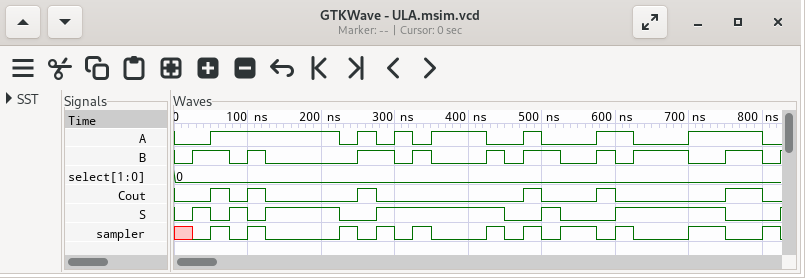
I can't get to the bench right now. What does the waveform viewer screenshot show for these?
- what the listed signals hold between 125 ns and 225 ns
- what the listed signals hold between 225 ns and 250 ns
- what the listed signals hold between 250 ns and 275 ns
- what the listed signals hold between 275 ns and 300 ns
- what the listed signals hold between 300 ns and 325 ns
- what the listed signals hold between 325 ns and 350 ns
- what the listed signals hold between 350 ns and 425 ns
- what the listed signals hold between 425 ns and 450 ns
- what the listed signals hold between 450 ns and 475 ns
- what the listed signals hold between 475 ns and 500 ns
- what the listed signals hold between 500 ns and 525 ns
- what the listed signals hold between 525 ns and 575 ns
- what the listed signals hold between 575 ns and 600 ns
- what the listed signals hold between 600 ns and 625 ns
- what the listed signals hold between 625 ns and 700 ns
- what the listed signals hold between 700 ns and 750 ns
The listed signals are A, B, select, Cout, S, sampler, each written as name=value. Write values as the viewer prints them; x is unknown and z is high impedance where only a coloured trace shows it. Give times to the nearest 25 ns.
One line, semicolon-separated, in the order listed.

A=1, B=0, select=0, Cout=0, S=1, sampler=0; A=0, B=0, select=0, Cout=0, S=0, sampler=1; A=1, B=1, select=0, Cout=1, S=0, sampler=0; A=0, B=1, select=0, Cout=0, S=1, sampler=1; A=1, B=0, select=0, Cout=0, S=1, sampler=0; A=0, B=1, select=0, Cout=0, S=1, sampler=1; A=1, B=0, select=0, Cout=0, S=1, sampler=0; A=0, B=1, select=0, Cout=0, S=1, sampler=1; A=0, B=0, select=0, Cout=0, S=0, sampler=0; A=1, B=1, select=0, Cout=1, S=0, sampler=1; A=0, B=1, select=0, Cout=0, S=1, sampler=0; A=0, B=0, select=0, Cout=0, S=0, sampler=1; A=1, B=1, select=0, Cout=1, S=0, sampler=0; A=1, B=0, select=0, Cout=0, S=1, sampler=1; A=0, B=1, select=0, Cout=0, S=1, sampler=0; A=1, B=0, select=0, Cout=0, S=1, sampler=1
